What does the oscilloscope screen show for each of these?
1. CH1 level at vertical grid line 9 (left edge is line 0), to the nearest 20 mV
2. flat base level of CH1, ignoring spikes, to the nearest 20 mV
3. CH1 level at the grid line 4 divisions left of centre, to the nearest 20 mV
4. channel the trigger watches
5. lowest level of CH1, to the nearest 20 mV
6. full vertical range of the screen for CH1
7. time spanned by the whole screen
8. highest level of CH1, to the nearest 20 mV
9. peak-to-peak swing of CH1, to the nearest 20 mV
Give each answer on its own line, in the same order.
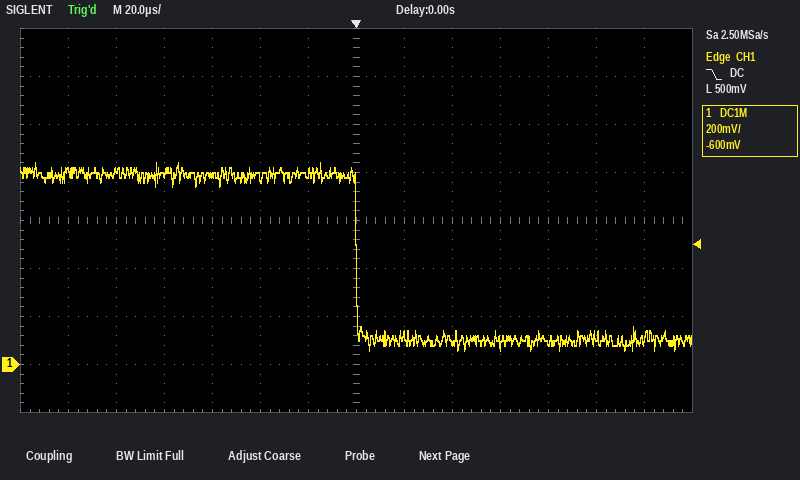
100 mV
100 mV
800 mV
CH1
60 mV
1.6 V
280 µs
840 mV
780 mV
